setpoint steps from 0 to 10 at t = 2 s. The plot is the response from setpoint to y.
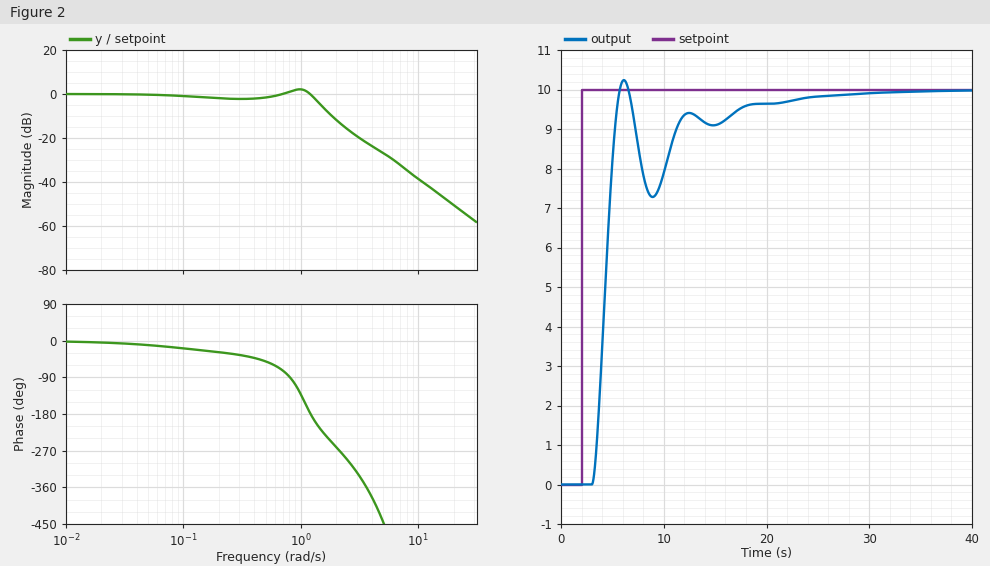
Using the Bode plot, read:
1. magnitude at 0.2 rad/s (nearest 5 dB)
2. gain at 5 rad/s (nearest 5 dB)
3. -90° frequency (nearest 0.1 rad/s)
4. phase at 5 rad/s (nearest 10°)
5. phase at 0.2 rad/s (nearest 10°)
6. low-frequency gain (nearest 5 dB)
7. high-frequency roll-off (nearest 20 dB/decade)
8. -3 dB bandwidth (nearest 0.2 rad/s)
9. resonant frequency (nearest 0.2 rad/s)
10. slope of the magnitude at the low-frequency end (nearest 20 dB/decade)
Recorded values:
0 dB
-25 dB
0.8 rad/s
-440°
-30°
0 dB
-40 dB/decade
1.4 rad/s
1.0 rad/s
0 dB/decade
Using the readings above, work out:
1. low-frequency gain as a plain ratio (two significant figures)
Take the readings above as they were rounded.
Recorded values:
1.0
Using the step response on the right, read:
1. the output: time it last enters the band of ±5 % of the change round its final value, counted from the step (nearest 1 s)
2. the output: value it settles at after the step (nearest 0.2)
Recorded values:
15 s
10.0
